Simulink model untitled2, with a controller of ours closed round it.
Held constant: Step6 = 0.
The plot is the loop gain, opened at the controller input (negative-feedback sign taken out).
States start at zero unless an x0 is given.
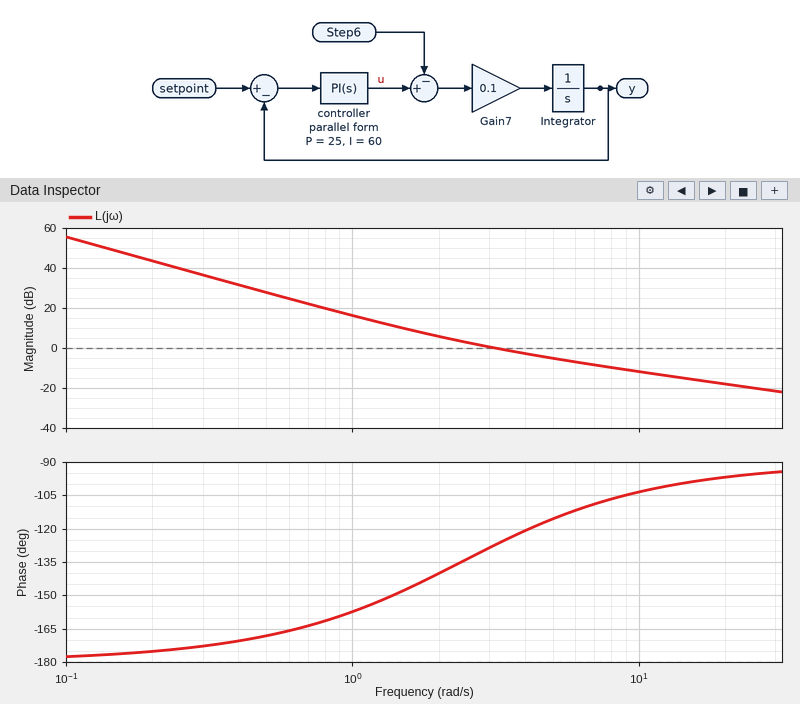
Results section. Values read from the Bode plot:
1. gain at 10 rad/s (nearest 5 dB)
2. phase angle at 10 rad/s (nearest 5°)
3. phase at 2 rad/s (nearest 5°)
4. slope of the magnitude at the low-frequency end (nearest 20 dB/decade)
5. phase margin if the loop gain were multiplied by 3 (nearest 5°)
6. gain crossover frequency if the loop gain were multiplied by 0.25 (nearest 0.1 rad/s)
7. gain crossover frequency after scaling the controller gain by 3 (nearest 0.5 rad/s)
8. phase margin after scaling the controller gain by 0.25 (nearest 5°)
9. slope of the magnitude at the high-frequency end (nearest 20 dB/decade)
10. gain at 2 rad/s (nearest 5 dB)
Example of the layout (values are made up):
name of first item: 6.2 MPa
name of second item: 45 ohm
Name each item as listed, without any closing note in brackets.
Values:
gain at 10 rad/s: -10 dB
phase angle at 10 rad/s: -105°
phase at 2 rad/s: -140°
slope of the magnitude at the low-frequency end: -40 dB/decade
phase margin if the loop gain were multiplied by 3: 75°
gain crossover frequency if the loop gain were multiplied by 0.25: 1.3 rad/s
gain crossover frequency after scaling the controller gain by 3: 8.0 rad/s
phase margin after scaling the controller gain by 0.25: 30°
slope of the magnitude at the high-frequency end: -20 dB/decade
gain at 2 rad/s: 5 dB
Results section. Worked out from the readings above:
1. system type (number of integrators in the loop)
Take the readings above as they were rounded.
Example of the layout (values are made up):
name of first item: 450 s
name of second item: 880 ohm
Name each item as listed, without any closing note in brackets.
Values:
system type: 2
